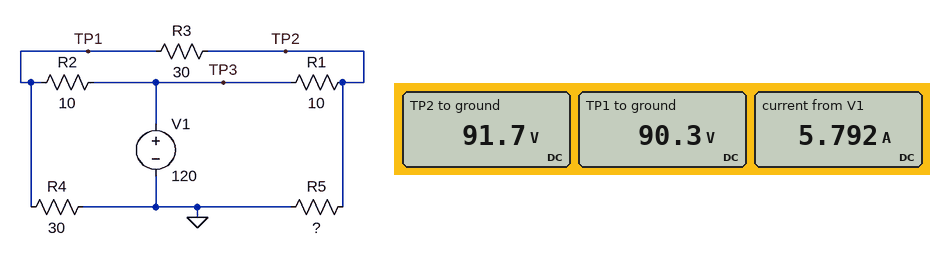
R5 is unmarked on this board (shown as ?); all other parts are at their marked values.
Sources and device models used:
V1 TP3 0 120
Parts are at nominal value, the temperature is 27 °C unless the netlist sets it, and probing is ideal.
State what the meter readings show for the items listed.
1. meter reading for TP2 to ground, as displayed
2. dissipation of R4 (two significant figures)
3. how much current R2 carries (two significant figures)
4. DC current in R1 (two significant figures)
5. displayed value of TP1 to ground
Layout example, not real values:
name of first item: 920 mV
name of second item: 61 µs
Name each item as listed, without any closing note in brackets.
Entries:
meter reading for TP2 to ground, as displayed: 91.7 V
dissipation of R4: 270 W
how much current R2 carries: 3.0 A
DC current in R1: 2.8 A
displayed value of TP1 to ground: 90.3 V
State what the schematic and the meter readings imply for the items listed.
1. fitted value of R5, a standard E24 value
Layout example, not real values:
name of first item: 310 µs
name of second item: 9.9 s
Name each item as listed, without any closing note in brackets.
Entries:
fitted value of R5, a standard E24 value: 33 Ω
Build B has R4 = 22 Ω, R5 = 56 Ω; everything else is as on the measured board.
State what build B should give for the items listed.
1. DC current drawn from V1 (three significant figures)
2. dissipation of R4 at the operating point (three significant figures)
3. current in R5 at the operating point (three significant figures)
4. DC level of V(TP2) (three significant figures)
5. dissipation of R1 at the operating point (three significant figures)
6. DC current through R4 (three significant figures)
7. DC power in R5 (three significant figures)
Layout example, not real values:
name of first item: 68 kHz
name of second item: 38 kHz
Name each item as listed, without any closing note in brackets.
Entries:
DC current drawn from V1: 5.64 A
dissipation of R4 at the operating point: 332 W
current in R5 at the operating point: 1.75 A
DC level of V(TP2): 98.2 V
dissipation of R1 at the operating point: 47.5 W
DC current through R4: 3.88 A
DC power in R5: 172 W
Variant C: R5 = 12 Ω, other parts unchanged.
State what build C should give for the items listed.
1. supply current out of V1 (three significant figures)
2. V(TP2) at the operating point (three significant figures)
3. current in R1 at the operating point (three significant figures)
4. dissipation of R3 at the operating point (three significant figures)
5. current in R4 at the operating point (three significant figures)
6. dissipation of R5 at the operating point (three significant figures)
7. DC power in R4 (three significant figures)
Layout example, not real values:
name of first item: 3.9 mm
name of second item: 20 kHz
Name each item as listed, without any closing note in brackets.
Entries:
supply current out of V1: 8.57 A
V(TP2) at the operating point: 68.6 V
current in R1 at the operating point: 5.14 A
dissipation of R3 at the operating point: 9.80 W
current in R4 at the operating point: 2.86 A
dissipation of R5 at the operating point: 392 W
DC power in R4: 245 W
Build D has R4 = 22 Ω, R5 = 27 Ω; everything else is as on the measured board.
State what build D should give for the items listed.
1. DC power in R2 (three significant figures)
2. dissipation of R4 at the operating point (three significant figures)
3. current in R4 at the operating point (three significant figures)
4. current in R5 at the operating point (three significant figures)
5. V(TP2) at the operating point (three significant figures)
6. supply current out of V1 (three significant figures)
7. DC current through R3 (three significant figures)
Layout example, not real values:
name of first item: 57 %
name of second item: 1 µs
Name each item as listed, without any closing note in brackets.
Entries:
DC power in R2: 135 W
dissipation of R4 at the operating point: 315 W
current in R4 at the operating point: 3.79 A
current in R5 at the operating point: 3.21 A
V(TP2) at the operating point: 86.7 V
supply current out of V1: 7.00 A
DC current through R3: 115 mA
